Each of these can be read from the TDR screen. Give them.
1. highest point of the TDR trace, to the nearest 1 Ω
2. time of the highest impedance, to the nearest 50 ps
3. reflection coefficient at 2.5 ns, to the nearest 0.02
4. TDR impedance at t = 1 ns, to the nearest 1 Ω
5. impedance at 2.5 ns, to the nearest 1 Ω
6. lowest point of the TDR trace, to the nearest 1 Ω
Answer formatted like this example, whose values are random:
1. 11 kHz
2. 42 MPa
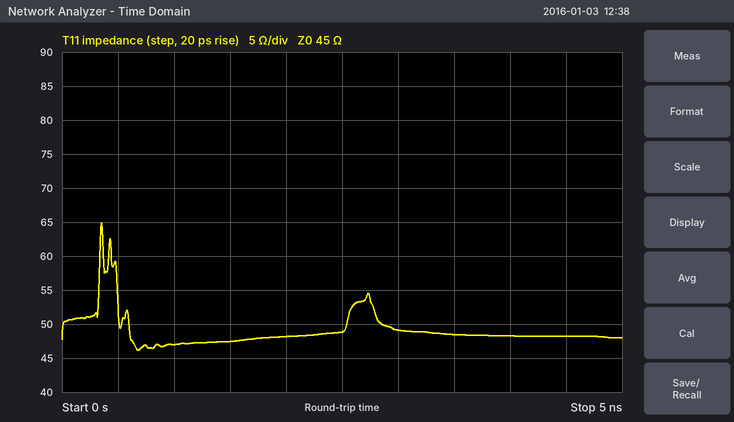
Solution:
1. 65 Ω
2. 350 ps
3. +0.04
4. 47 Ω
5. 49 Ω
6. 46 Ω
